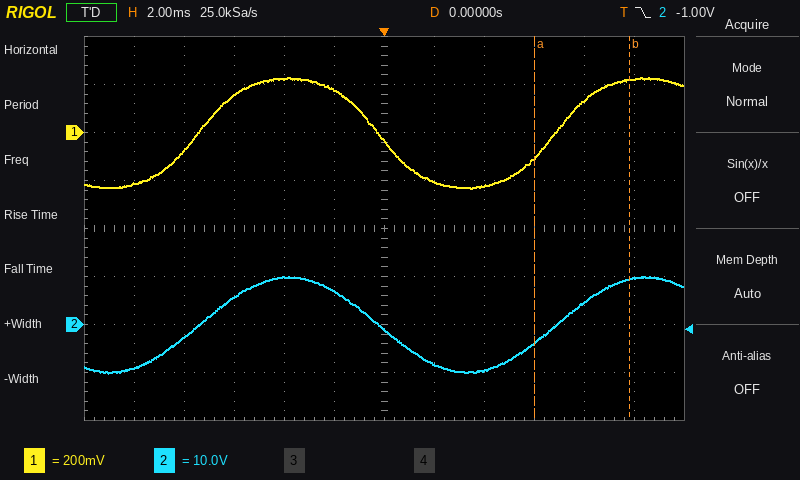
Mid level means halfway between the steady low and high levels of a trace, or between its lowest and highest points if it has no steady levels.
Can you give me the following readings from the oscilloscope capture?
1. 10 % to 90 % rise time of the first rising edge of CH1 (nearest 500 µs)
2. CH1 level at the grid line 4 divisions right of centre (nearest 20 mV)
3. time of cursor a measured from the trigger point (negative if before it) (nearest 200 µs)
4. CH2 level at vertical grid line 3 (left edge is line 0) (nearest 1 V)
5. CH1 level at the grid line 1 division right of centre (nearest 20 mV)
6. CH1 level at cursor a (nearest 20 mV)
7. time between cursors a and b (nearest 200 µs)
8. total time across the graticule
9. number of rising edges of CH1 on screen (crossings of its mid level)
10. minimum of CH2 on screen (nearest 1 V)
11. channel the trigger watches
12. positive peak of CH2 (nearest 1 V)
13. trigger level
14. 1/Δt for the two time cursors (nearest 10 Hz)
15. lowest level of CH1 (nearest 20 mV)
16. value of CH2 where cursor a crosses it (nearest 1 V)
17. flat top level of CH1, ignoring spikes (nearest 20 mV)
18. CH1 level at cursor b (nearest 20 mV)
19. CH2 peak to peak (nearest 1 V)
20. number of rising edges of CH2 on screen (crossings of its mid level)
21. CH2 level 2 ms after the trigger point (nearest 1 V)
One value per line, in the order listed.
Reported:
3.5 ms
140 mV
+6.0 ms
6 V
-200 mV
-100 mV
3.8 ms
24 ms
2
-10 V
CH2
10 V
-1.00 V
260 Hz
-240 mV
-4 V
220 mV
220 mV
20 V
2
-8 V
